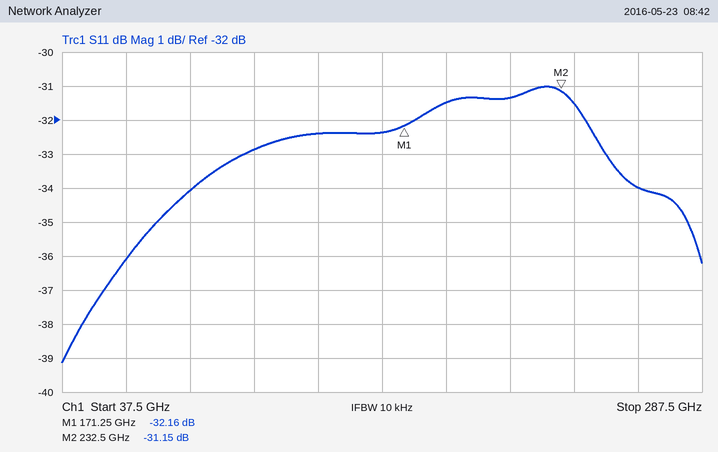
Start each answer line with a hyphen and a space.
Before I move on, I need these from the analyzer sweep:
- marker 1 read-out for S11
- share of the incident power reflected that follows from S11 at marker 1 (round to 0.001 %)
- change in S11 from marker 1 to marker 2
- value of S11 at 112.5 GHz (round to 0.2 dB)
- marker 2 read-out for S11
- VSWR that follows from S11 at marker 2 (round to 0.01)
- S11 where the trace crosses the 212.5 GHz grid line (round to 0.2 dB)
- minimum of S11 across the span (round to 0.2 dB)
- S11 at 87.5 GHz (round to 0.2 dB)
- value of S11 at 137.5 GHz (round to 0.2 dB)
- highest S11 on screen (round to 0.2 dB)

- -32.16 dB
- 0.061 %
- 1.01 dB
- -32.8 dB
- -31.15 dB
- 1.06
- -31.4 dB
- -39.2 dB
- -34.0 dB
- -32.4 dB
- -31.0 dB
